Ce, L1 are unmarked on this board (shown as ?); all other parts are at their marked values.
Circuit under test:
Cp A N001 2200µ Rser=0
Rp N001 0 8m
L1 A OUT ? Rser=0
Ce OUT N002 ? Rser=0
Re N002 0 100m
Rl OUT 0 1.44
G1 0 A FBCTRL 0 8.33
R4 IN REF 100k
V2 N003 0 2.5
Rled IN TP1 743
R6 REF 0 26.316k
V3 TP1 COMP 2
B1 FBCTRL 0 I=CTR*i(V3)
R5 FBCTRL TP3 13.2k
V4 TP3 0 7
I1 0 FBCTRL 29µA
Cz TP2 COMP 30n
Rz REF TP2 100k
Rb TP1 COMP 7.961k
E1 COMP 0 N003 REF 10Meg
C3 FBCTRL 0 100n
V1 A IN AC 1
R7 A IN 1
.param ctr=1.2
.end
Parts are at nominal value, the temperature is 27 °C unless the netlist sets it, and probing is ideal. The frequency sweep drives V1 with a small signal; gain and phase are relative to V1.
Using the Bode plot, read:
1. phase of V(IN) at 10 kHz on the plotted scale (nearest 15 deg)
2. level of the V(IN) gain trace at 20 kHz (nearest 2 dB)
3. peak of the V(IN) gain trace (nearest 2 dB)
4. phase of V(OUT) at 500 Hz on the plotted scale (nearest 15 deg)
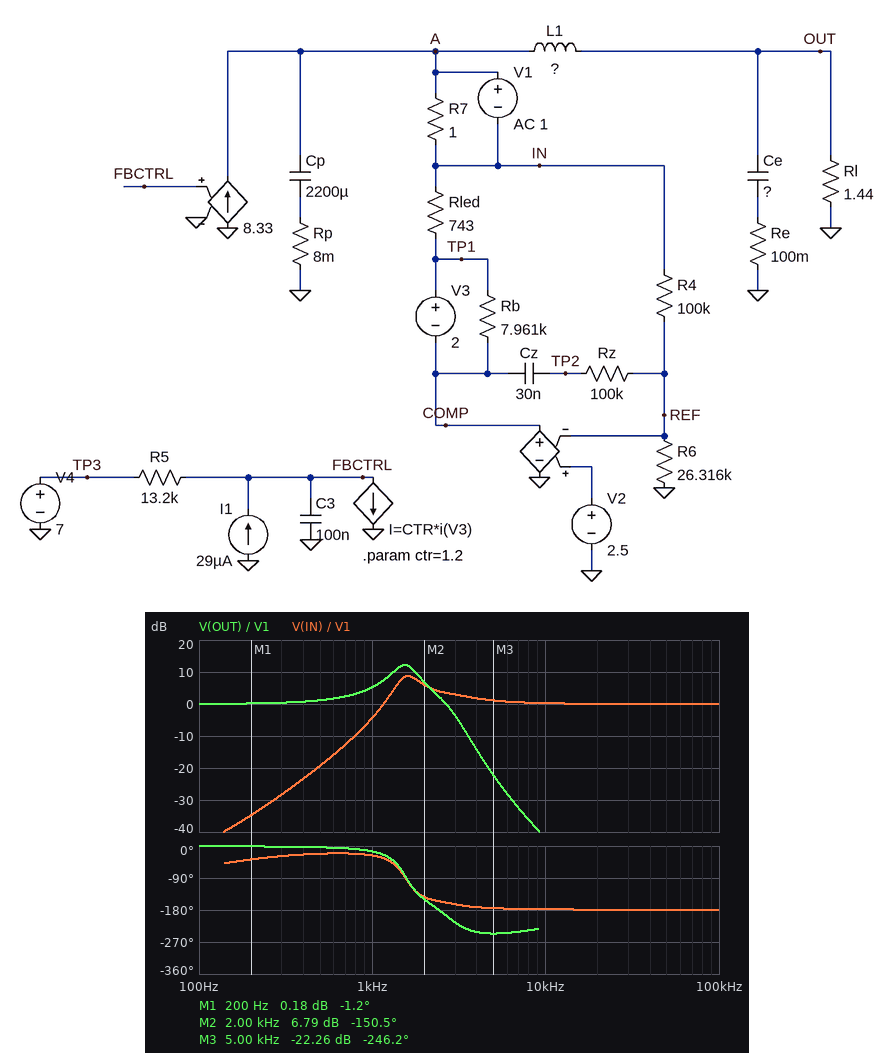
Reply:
-180 deg
0 dB
8 dB
0 deg
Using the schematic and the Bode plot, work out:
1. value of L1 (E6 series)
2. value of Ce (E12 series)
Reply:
10 µH
390 µF
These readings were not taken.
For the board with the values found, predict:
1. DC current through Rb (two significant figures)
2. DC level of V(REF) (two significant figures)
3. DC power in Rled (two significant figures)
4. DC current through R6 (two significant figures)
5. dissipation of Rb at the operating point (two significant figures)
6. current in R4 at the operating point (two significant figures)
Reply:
250 µA
2.5 V
320 µW
95 µA
500 µW
95 µA
